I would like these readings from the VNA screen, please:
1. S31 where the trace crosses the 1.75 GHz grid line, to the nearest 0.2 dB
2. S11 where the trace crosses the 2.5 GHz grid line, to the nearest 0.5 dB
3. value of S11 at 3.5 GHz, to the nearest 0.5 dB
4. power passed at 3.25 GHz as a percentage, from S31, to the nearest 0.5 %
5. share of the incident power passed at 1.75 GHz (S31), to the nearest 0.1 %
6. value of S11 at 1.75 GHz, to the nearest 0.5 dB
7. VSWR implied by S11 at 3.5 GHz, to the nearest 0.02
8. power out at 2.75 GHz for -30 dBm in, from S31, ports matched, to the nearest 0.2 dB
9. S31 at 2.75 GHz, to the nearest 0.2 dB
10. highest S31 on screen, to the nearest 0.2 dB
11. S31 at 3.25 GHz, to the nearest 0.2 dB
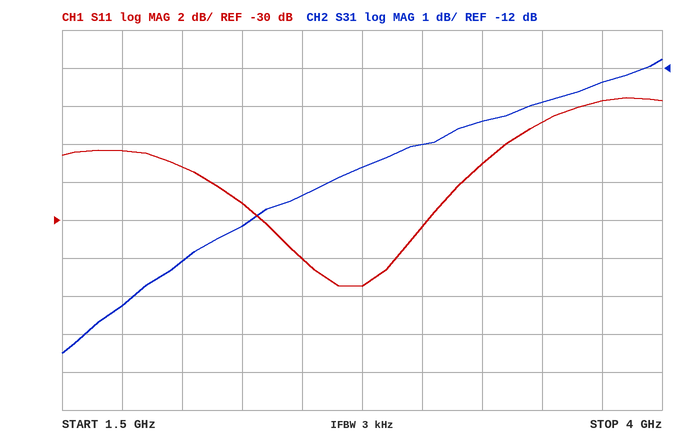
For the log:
-18.2 dB
-32.0 dB
-25.0 dB
4.5 %
1.5 %
-26.5 dB
1.12
-44.6 dBm
-14.6 dB
-11.8 dB
-13.4 dB
